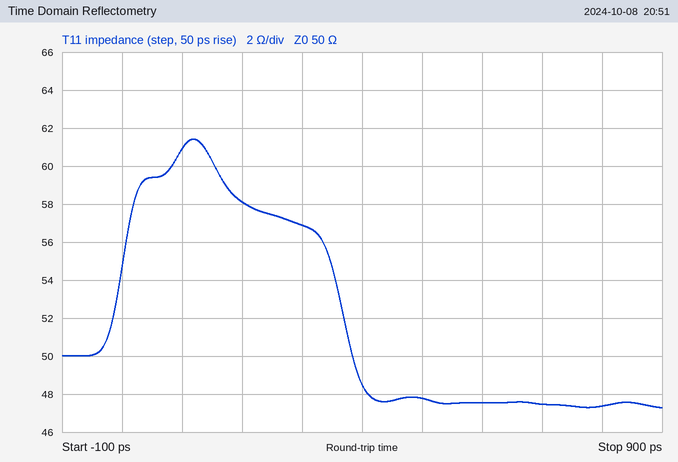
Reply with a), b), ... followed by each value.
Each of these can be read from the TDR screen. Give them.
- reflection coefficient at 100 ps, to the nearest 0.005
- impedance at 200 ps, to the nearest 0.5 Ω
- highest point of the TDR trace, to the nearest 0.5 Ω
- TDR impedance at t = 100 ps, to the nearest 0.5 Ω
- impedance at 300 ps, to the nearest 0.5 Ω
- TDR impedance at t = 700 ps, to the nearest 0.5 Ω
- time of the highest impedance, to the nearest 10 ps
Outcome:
a) +0.100
b) 58.0 Ω
c) 61.5 Ω
d) 61.0 Ω
e) 57.0 Ω
f) 47.5 Ω
g) 120 ps
